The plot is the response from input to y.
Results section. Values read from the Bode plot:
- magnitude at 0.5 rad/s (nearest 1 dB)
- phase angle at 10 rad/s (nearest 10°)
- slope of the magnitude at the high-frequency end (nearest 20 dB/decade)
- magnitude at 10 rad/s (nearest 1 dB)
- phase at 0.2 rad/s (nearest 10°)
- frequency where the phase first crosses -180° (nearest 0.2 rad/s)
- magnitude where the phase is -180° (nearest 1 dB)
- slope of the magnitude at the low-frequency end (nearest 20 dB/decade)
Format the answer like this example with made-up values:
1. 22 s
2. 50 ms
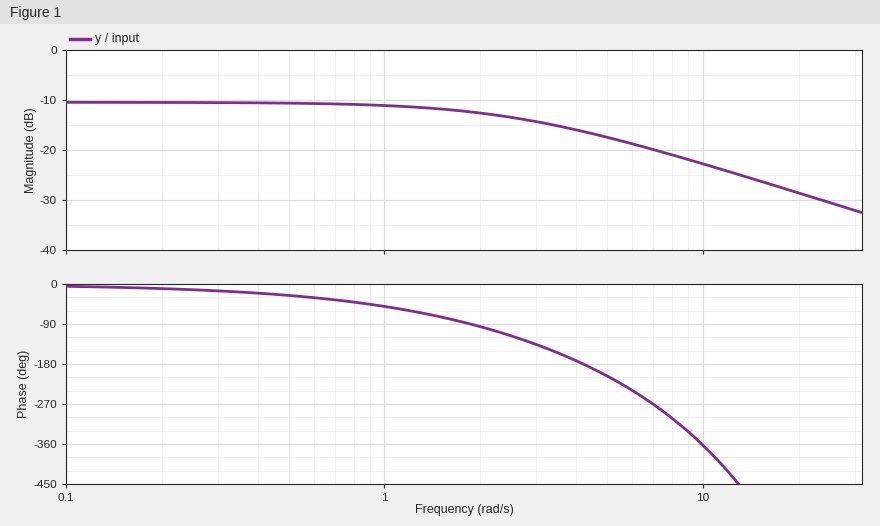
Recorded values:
1. -11 dB
2. -360°
3. -20 dB/decade
4. -23 dB
5. -10°
6. 4.2 rad/s
7. -16 dB
8. 0 dB/decade
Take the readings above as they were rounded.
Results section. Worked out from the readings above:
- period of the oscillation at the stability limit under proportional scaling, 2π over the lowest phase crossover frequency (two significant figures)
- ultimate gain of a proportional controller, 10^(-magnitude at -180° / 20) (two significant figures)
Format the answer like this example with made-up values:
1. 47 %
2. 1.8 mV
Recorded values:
1. 1.5 s
2. 6.3
